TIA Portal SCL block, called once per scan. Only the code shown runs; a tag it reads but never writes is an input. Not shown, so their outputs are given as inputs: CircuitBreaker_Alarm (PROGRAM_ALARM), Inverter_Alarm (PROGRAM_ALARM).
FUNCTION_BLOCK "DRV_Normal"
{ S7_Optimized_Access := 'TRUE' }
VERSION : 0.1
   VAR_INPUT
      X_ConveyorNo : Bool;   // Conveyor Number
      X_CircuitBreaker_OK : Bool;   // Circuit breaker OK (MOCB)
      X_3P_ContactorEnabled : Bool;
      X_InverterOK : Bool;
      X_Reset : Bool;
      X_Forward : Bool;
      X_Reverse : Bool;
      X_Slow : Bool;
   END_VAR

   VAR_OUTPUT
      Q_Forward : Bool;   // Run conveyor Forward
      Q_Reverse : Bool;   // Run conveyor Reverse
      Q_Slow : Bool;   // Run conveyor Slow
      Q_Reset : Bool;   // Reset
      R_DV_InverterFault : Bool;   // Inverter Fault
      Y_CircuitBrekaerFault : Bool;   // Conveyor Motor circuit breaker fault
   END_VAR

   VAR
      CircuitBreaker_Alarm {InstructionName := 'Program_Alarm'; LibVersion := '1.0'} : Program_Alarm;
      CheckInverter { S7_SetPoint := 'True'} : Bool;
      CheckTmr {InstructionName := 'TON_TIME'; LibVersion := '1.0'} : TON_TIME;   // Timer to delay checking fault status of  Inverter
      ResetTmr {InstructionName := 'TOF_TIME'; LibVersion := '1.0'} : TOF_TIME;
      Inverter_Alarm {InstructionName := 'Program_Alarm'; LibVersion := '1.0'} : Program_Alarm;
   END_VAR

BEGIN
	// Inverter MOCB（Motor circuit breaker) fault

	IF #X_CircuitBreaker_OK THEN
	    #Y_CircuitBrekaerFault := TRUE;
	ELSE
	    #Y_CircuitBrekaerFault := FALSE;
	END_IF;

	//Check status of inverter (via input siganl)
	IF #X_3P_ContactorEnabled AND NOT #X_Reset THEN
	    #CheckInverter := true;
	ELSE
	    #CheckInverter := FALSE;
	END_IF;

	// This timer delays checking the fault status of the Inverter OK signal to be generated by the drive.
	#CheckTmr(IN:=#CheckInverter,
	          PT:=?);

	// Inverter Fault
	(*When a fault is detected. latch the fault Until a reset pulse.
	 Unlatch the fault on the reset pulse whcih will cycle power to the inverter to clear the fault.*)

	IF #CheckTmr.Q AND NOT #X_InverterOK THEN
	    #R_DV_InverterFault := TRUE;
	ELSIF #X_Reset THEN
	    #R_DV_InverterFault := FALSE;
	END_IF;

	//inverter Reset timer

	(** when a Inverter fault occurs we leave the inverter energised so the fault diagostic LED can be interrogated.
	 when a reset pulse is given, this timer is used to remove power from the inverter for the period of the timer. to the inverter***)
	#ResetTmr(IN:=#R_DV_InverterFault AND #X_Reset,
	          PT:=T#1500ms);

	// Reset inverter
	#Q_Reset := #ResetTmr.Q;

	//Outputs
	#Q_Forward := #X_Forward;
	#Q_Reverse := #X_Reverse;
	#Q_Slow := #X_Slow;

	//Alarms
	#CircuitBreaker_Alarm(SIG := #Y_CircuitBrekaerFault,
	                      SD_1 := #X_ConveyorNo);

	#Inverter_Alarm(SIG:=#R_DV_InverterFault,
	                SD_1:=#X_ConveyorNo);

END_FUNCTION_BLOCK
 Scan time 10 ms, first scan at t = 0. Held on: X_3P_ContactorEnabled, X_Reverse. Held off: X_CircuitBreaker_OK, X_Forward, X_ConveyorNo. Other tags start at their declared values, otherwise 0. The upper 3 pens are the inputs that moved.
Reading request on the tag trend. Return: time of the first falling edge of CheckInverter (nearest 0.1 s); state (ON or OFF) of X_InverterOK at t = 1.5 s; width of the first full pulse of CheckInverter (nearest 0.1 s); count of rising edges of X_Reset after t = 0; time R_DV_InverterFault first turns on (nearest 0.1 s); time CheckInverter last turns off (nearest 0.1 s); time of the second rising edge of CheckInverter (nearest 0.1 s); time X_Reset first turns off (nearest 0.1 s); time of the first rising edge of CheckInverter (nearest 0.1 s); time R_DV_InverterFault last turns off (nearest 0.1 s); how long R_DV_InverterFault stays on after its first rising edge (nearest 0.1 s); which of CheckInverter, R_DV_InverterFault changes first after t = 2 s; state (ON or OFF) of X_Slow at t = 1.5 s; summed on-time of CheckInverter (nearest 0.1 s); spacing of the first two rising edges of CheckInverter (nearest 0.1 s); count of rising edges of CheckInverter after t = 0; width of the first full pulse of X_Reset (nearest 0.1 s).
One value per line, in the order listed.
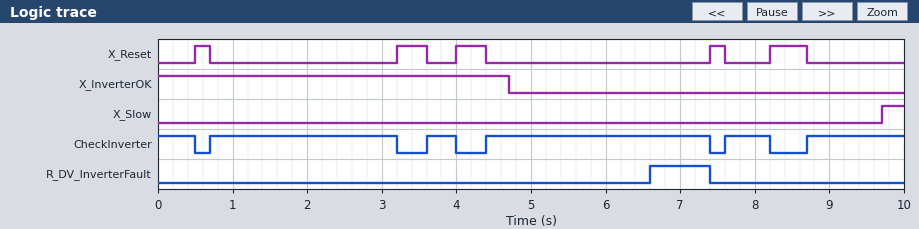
0.5 s
ON
2.5 s
5
6.6 s
8.2 s
3.6 s
0.7 s
0.7 s
7.4 s
0.8 s
CheckInverter
OFF
8.3 s
2.9 s
5
0.2 s
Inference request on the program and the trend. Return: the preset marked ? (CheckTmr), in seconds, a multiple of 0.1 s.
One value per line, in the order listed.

2.2 s
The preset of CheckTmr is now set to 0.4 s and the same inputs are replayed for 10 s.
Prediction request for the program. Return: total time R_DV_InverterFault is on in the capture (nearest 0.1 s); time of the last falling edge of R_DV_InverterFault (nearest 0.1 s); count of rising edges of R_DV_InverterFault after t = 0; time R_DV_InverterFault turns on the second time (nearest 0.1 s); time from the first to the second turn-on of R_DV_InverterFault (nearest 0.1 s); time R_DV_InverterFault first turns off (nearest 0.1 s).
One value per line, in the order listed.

3.7 s
8.2 s
3
8.0 s
3.2 s
7.4 s
